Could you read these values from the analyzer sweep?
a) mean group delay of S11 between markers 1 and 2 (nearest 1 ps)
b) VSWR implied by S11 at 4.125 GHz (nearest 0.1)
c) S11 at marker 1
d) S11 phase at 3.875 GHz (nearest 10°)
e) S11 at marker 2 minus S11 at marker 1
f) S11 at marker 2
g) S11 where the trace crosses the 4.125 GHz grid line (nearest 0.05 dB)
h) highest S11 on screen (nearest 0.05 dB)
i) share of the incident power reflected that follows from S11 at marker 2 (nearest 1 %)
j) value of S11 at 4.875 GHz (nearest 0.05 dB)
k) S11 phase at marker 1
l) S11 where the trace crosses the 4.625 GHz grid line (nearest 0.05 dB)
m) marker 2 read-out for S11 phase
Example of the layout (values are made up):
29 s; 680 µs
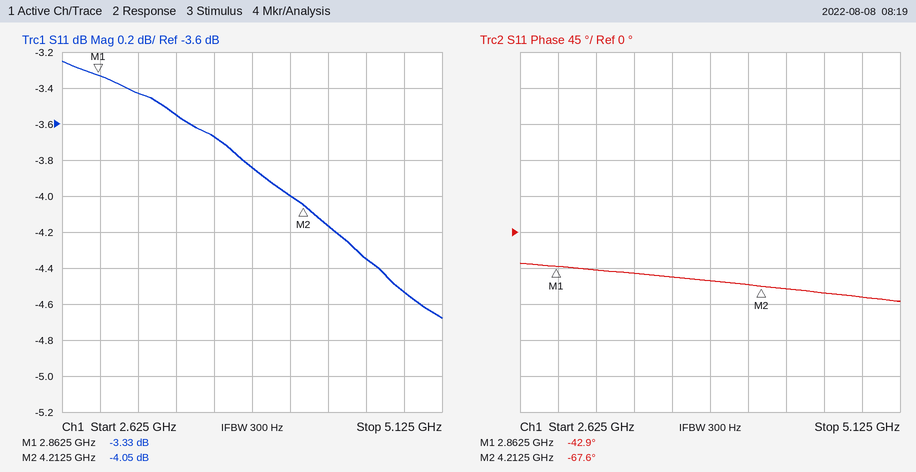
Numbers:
51 ps; 4.4; -3.33 dB; -60°; -0.72 dB; -4.05 dB; -4.00 dB; -3.25 dB; 39 %; -4.55 dB; -42.9°; -4.35 dB; -67.6°
